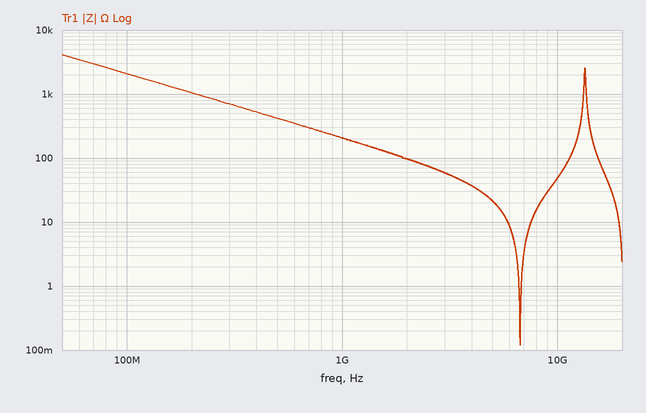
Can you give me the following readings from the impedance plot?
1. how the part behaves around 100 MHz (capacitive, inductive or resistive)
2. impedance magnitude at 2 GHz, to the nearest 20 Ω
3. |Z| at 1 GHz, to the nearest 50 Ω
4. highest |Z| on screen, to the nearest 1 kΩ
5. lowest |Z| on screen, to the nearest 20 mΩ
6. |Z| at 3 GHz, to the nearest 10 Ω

capacitive
100 Ω
200 Ω
4 kΩ
120 mΩ
60 Ω
